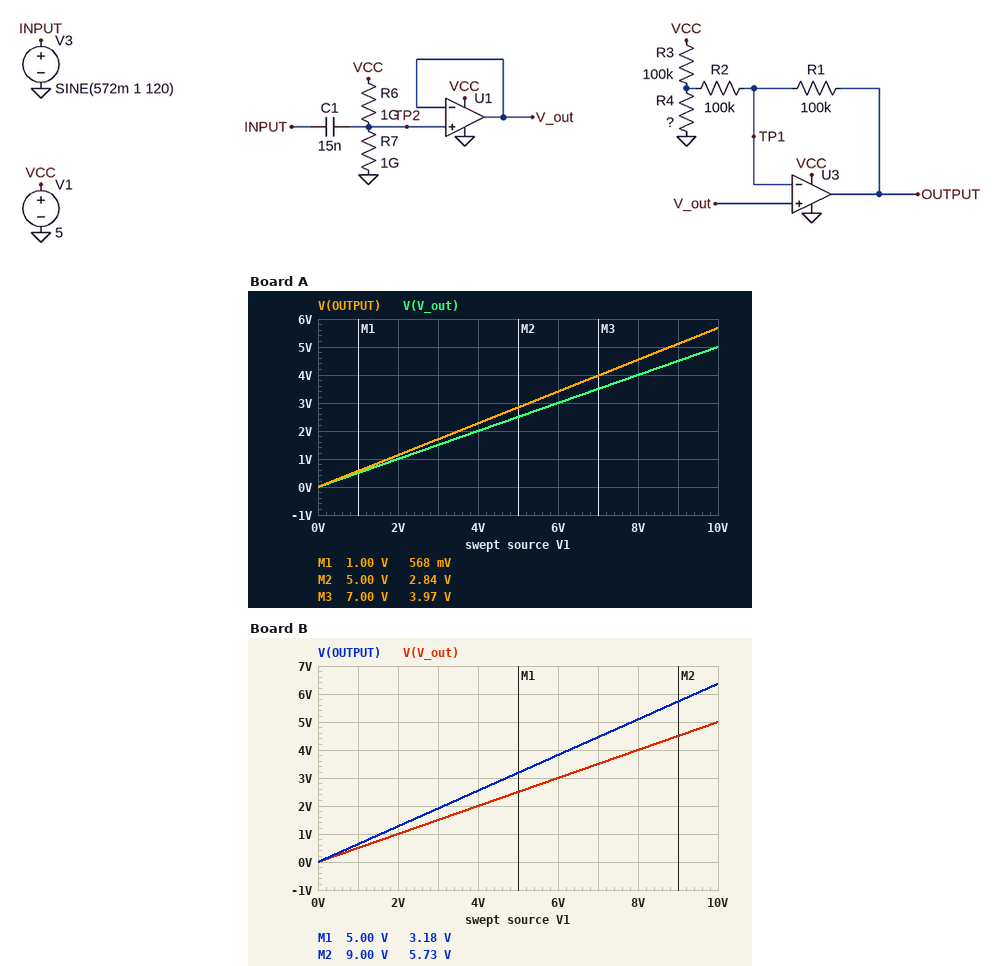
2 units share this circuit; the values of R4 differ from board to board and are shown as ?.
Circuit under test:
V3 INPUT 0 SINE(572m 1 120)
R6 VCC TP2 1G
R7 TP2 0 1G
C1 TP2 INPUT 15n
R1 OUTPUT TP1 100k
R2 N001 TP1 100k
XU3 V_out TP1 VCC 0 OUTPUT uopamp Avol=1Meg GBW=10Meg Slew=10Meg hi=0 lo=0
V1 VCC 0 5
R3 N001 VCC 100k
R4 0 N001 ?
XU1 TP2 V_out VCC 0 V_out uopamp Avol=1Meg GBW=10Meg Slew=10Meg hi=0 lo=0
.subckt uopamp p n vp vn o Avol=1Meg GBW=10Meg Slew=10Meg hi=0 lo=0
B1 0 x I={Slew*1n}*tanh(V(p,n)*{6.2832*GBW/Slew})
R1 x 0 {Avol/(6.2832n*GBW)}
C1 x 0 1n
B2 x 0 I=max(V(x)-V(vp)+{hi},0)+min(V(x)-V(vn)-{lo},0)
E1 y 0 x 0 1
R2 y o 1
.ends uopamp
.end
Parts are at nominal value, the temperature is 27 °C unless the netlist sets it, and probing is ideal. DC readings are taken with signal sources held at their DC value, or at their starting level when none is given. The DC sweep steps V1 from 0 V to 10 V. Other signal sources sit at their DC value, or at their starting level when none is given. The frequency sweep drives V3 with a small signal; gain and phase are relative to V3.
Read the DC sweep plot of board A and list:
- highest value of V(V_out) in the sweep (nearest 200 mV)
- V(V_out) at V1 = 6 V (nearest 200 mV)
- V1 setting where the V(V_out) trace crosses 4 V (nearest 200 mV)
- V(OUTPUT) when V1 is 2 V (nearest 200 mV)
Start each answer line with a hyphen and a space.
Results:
- 5.0 V
- 3.0 V
- 8.0 V
- 1.2 V
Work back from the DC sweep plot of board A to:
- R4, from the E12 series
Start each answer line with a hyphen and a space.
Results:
- 68 kΩ
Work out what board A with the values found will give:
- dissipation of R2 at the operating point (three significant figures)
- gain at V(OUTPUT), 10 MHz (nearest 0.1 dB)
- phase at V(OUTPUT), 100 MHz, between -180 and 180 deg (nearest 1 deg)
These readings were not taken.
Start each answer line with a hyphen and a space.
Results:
- 1.15 µW
- -4.3 dB
- -171 deg
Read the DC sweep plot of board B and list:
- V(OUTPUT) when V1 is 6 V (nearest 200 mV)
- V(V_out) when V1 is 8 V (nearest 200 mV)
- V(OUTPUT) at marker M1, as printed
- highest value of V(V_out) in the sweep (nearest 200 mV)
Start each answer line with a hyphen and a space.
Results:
- 3.8 V
- 4.0 V
- 3.18 V
- 5.0 V
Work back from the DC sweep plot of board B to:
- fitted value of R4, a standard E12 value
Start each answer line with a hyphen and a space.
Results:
- 47 kΩ
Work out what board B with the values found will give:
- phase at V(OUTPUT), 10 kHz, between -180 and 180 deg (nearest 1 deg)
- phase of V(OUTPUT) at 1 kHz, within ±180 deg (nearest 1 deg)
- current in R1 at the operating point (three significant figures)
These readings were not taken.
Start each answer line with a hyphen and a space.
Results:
- 0 deg
- 0 deg
- 6.83 µA
